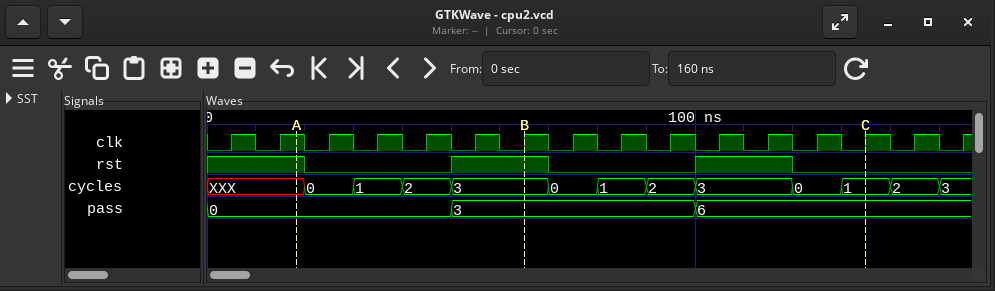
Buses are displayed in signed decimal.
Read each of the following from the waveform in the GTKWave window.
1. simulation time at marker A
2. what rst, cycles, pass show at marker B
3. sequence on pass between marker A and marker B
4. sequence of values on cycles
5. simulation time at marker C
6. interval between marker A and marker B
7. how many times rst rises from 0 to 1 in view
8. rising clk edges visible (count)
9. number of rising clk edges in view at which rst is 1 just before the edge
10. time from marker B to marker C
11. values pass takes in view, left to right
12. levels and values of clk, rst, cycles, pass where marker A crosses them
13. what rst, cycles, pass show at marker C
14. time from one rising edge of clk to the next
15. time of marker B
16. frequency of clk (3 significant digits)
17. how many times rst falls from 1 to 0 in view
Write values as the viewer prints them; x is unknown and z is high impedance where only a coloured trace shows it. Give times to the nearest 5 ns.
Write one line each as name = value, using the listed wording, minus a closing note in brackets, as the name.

simulation time at marker A = 20 ns
what rst, cycles, pass show at marker B = rst=1, cycles=3, pass=3
sequence on pass between marker A and marker B = 0, 3
sequence of values on cycles = XXX, 0, 1, 2, 3, 0, 1, 2, 3, 0, 1, 2, 3
simulation time at marker C = 135 ns
interval between marker A and marker B = 45 ns
how many times rst rises from 0 to 1 in view = 2
rising clk edges visible = 16
number of rising clk edges in view at which rst is 1 just before the edge = 6
time from marker B to marker C = 70 ns
values pass takes in view, left to right = 0, 3, 6
levels and values of clk, rst, cycles, pass where marker A crosses them = clk=1, rst=1, cycles=XXX, pass=0
what rst, cycles, pass show at marker C = rst=0, cycles=1, pass=6
time from one rising edge of clk to the next = 10 ns
time of marker B = 65 ns
frequency of clk = 100 MHz
how many times rst falls from 1 to 0 in view = 3
